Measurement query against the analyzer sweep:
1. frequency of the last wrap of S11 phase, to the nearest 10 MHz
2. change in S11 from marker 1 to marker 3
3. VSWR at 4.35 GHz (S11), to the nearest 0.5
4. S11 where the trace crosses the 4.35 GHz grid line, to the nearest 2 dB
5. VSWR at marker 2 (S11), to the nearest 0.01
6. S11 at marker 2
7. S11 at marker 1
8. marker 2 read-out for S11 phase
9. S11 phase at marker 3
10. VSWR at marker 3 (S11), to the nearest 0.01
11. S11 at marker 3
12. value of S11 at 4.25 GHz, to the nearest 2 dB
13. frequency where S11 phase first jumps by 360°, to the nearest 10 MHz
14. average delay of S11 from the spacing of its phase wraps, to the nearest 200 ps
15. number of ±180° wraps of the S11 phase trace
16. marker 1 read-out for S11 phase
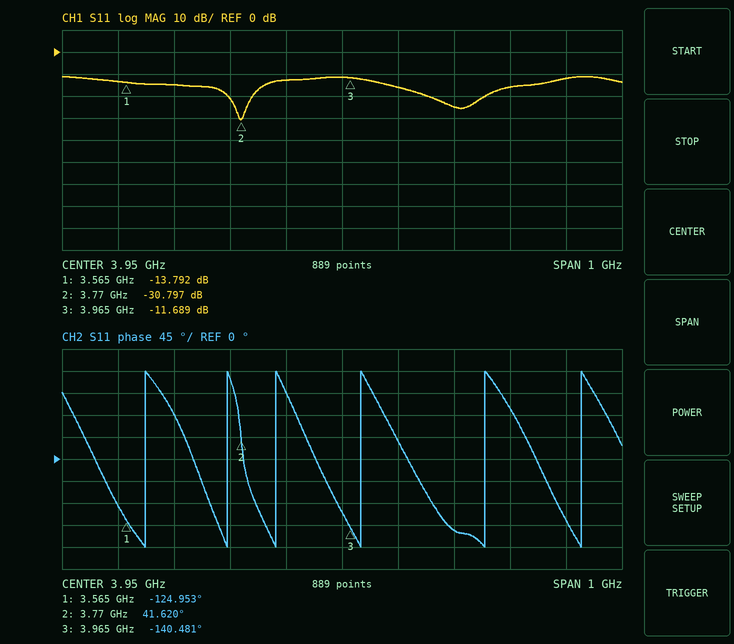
4.38 GHz
2.103 dB
1.5
-12 dB
1.06
-30.797 dB
-13.792 dB
41.620°
-140.481°
1.70
-11.689 dB
-16 dB
3.60 GHz
6.4 ns
6
-124.953°
